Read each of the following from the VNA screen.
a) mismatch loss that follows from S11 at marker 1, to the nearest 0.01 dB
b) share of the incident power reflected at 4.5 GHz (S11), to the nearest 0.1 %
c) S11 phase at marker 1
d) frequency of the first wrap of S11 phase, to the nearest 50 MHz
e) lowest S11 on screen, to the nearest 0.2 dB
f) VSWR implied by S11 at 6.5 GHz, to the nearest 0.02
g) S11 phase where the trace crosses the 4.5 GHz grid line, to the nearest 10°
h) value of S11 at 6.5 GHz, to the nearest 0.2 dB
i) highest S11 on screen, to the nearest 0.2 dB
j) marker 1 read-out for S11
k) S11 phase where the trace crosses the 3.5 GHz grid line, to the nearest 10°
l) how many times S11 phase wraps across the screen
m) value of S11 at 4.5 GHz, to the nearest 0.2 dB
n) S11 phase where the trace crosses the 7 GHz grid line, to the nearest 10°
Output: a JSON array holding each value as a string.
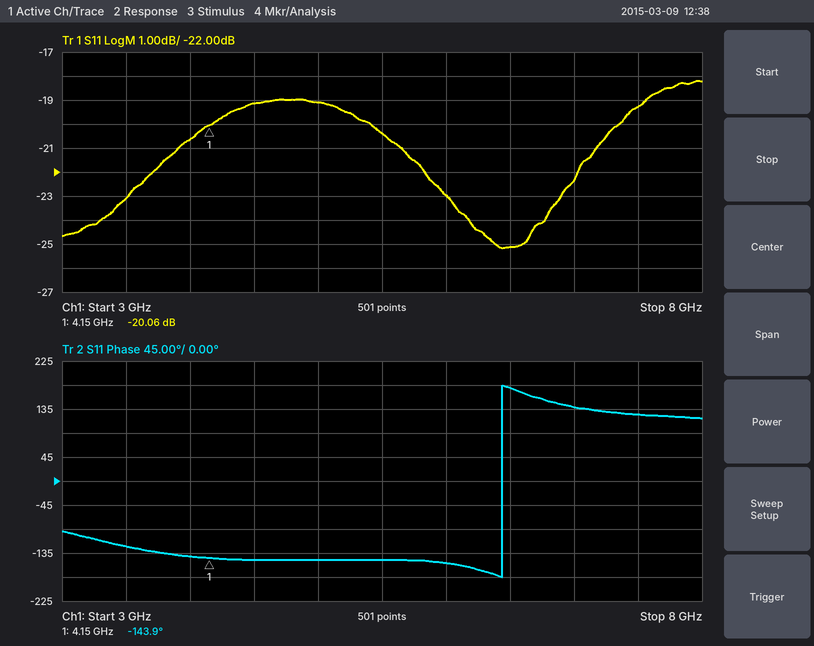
["0.04 dB", "1.2 %", "-143.9°", "6.45 GHz", "-25.2 dB", "1.12", "-150°", "-25.2 dB", "-18.2 dB", "-20.06 dB", "-120°", "1", "-19.2 dB", "140°"]
